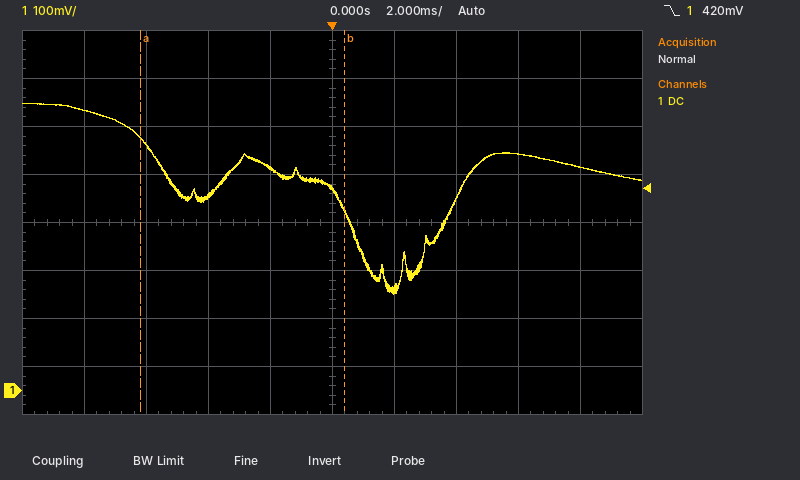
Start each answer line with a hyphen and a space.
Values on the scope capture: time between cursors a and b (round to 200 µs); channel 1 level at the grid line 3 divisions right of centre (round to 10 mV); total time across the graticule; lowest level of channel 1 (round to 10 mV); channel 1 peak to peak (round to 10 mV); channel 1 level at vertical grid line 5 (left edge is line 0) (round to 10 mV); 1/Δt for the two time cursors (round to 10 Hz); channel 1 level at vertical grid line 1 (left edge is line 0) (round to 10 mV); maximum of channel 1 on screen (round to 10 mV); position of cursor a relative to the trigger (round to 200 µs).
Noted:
- 6.6 ms
- 490 mV
- 20 ms
- 200 mV
- 400 mV
- 420 mV
- 150 Hz
- 580 mV
- 600 mV
- -6.2 ms
